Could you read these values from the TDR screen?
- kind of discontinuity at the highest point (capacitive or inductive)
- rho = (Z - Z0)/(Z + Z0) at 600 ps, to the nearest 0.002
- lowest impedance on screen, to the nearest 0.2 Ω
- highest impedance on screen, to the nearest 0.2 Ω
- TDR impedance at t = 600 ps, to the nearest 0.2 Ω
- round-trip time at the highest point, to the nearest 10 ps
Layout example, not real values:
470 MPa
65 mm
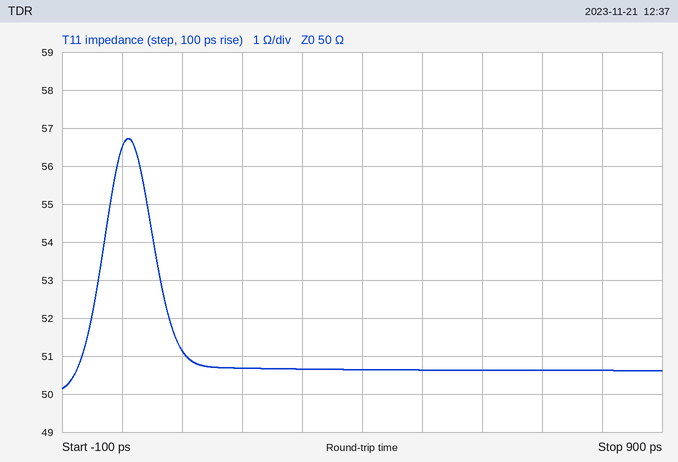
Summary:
inductive
+0.006
50.2 Ω
56.8 Ω
50.6 Ω
10 ps
